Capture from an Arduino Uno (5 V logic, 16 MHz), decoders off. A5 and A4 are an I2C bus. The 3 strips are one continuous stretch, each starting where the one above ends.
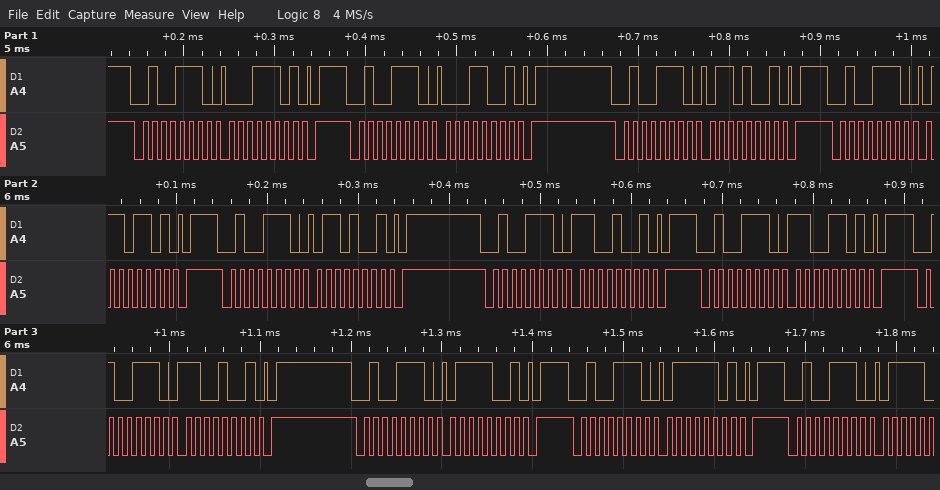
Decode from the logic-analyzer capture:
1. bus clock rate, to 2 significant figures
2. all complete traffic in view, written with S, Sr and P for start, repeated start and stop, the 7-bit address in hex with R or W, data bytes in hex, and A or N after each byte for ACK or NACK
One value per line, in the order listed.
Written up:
100 kHz
S 27W A 1D A P S 27W A 19 A P S 27W A 69 A P S 27W A 6D A P S 27W A 69 A P S 27W A C9 A P S 27W A CD A P S 27W A C9 A P S 27W A 79 A P S 27W A 7D A P S 27W A
